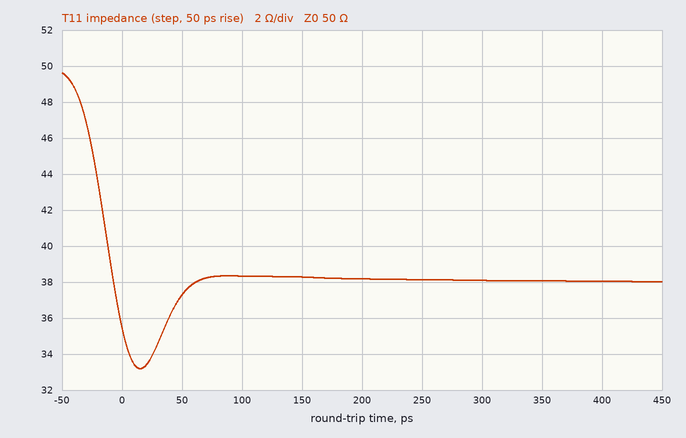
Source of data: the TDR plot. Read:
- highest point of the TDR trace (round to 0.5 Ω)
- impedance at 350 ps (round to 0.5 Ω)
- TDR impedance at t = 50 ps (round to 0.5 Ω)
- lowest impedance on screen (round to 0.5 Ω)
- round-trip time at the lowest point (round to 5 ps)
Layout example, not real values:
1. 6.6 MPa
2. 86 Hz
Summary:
1. 49.5 Ω
2. 38.0 Ω
3. 37.5 Ω
4. 33.0 Ω
5. 15 ps
